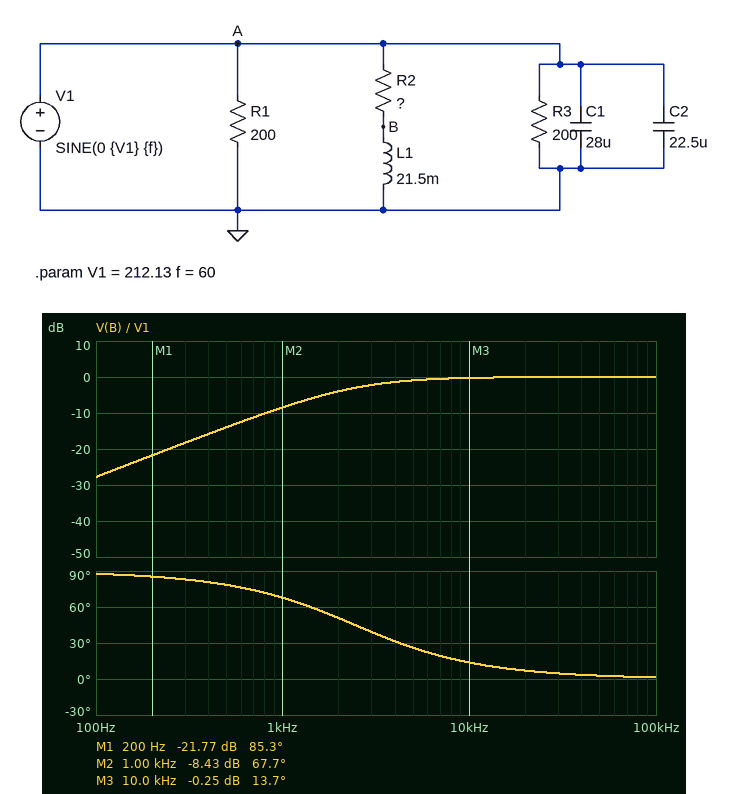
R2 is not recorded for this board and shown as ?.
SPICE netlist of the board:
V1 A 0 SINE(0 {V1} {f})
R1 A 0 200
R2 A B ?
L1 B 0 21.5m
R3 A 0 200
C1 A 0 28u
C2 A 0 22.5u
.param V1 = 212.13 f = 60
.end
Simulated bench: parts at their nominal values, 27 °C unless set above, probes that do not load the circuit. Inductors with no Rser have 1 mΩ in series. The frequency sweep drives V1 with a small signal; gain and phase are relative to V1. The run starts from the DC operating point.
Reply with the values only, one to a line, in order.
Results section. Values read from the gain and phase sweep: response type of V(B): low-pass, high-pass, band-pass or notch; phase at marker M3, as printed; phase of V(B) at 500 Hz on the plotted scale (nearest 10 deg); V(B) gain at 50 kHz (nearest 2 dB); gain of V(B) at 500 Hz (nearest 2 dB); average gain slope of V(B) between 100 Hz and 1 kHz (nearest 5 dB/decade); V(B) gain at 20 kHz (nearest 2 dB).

high-pass
13.7 deg
80 deg
0 dB
-14 dB
20 dB/decade
0 dB
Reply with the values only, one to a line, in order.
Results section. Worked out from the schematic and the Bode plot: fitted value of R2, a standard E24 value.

330 Ω
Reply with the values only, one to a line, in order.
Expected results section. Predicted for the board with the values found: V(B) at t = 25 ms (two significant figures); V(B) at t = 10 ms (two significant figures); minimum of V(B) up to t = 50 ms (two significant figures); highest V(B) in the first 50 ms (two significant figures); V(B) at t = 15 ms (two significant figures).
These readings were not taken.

-5.2 V
-4.3 V
-5.2 V
5.2 V
4.1 V
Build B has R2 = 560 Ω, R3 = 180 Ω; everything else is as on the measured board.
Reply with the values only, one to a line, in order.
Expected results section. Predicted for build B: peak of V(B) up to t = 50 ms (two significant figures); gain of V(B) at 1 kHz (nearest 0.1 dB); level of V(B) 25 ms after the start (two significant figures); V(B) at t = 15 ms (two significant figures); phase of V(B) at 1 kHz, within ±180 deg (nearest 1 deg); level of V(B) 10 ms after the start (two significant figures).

3.1 V
-12.6 dB
-3.1 V
2.5 V
76 deg
-2.5 V
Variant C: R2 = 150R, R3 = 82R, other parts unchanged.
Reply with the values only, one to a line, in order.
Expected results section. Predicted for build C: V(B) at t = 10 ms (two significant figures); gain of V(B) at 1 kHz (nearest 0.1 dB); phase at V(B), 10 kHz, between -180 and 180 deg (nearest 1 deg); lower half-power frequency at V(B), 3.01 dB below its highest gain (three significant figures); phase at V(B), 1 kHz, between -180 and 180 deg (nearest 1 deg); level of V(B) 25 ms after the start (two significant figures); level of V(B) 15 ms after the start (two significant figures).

-9.6 V
-3.5 dB
6 deg
1.11 kHz
48 deg
-11 V
8.9 V
